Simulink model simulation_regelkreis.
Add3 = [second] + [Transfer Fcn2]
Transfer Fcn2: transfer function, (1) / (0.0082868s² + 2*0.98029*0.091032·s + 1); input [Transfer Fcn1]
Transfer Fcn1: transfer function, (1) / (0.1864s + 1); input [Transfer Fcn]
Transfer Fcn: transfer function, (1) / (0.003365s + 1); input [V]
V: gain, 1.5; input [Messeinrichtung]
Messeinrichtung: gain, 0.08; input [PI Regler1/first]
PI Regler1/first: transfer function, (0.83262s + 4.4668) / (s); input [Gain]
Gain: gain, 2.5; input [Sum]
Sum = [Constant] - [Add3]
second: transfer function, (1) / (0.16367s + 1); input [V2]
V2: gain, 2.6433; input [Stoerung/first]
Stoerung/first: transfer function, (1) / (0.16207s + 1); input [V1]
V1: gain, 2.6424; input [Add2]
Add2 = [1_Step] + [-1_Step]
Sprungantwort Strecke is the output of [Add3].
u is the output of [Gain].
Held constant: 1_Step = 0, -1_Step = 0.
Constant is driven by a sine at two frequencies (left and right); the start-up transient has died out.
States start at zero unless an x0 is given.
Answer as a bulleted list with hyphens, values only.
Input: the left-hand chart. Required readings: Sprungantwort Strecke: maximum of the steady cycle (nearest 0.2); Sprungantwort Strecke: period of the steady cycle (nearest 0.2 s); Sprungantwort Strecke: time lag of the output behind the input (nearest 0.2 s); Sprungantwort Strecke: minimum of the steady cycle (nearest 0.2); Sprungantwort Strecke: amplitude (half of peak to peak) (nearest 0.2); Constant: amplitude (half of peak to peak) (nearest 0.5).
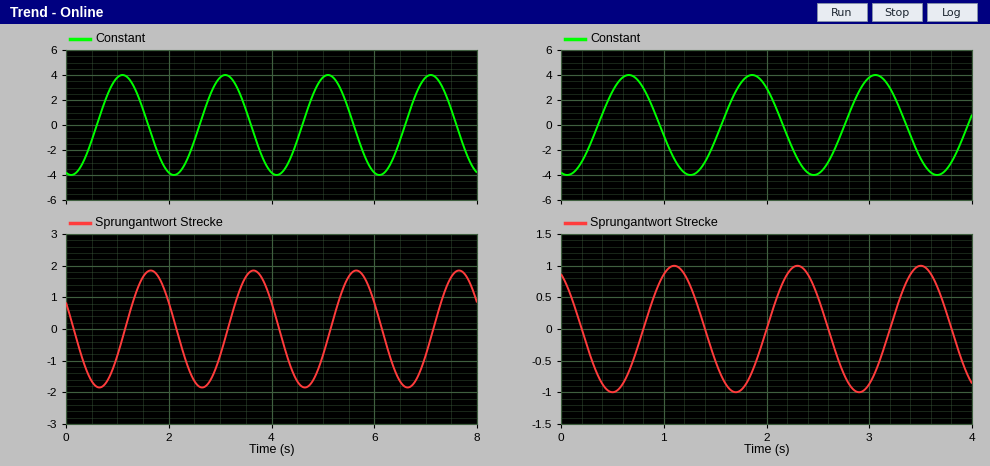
- 1.8
- 2.0 s
- 0.6 s
- -1.8
- 1.8
- 4.0
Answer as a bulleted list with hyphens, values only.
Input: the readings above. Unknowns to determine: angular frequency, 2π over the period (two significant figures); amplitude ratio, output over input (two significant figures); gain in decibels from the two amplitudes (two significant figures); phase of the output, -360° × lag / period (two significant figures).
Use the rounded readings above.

- 3.1 rad/s
- 0.45
- -6.9 dB
- -110°
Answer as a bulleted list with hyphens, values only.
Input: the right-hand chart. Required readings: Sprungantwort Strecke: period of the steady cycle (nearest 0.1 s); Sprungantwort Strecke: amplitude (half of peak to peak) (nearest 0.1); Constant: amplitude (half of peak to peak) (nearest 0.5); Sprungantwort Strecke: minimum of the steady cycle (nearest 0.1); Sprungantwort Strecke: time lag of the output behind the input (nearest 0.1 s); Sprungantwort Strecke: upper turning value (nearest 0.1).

- 1.2 s
- 1.0
- 4.0
- -1.0
- 0.4 s
- 1.0
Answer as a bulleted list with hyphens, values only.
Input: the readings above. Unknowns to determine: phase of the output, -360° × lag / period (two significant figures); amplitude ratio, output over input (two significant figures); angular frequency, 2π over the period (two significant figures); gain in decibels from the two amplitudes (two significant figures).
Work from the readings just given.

- -120°
- 0.25
- 5.2 rad/s
- -12 dB
